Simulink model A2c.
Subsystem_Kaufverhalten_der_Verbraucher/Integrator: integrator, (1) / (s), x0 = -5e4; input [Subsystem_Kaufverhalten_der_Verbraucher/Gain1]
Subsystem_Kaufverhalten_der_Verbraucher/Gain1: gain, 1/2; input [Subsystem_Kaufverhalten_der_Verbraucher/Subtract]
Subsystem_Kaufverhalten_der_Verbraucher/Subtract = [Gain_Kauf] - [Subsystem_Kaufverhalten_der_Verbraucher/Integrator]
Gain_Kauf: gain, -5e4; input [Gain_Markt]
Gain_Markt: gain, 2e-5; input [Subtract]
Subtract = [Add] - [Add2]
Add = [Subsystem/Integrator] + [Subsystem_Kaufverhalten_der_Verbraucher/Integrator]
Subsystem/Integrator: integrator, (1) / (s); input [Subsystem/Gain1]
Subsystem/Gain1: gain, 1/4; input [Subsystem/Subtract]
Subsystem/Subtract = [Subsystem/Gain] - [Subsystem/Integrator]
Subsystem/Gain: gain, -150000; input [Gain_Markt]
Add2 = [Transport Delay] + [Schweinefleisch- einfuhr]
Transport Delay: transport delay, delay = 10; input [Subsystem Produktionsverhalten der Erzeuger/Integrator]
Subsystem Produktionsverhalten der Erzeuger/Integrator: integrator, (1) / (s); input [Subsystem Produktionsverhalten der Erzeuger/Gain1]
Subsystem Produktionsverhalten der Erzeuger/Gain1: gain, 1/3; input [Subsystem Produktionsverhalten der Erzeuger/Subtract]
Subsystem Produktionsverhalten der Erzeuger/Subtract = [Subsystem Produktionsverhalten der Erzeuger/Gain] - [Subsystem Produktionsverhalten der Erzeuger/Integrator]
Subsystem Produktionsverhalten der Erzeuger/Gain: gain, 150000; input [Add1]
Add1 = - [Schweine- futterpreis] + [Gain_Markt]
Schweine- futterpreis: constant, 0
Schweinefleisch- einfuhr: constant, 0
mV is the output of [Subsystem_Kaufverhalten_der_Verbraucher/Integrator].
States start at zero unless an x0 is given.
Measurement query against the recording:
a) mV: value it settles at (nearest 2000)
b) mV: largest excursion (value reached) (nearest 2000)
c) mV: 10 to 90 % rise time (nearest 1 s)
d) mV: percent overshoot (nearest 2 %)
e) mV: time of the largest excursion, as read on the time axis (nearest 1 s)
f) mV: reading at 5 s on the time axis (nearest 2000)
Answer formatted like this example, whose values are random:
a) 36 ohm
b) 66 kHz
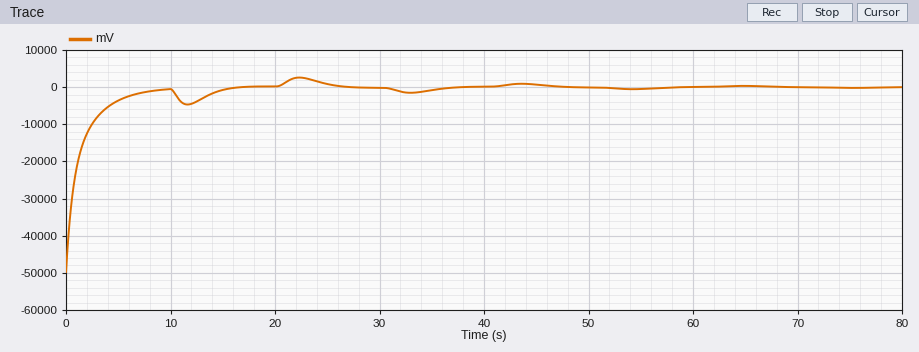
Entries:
a) 0
b) 2000
c) 4 s
d) 6 %
e) 22 s
f) -4000
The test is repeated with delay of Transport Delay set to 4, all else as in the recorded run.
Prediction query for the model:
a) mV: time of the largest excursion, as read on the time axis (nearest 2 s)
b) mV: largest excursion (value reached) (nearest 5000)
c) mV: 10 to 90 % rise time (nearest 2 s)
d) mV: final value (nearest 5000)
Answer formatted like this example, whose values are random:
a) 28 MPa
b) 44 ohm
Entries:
a) 10 s
b) 0
c) 6 s
d) 0
